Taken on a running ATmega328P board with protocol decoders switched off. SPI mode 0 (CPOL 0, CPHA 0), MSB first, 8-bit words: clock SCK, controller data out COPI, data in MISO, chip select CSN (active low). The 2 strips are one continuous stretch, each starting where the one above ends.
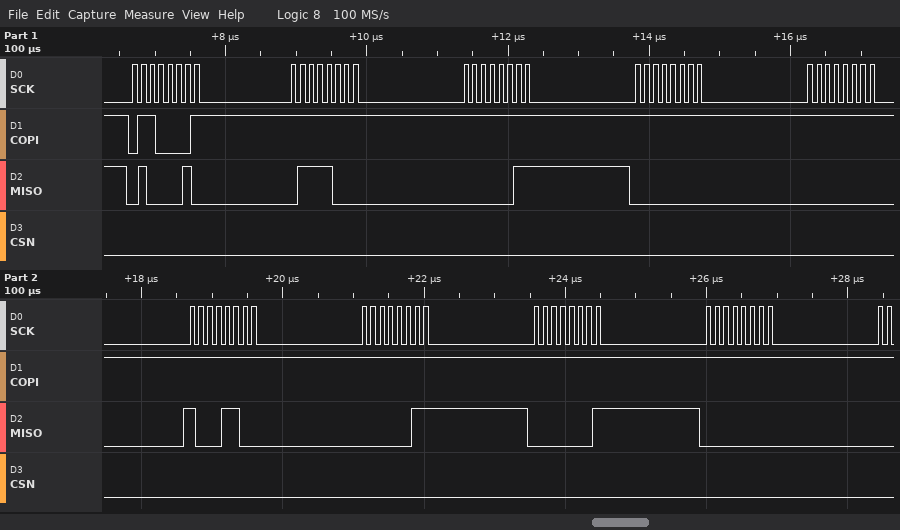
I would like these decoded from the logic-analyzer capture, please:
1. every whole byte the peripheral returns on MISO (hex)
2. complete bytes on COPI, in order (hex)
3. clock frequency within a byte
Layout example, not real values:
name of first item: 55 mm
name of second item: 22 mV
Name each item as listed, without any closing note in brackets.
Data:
every whole byte the peripheral returns on MISO: 42 78 03 00 00 8C 03 01 00
complete bytes on COPI, in order: 61 FF FF FF FF FF FF FF FF
clock frequency within a byte: 8 MHz
